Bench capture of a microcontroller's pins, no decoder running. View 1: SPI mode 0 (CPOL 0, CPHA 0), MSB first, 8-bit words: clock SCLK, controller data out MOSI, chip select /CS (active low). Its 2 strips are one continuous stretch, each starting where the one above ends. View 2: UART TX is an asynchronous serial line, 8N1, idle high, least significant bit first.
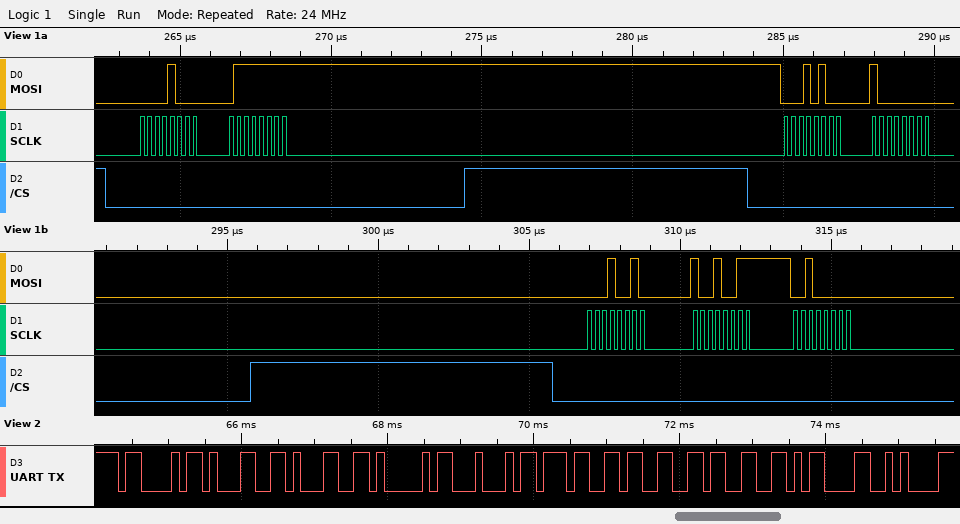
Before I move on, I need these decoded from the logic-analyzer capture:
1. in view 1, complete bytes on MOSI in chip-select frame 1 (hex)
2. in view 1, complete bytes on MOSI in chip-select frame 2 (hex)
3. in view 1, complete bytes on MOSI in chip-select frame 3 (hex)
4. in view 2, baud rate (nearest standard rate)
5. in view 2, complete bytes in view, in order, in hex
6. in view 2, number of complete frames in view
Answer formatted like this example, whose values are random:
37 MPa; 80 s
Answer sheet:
0x08 0x7F; 0x14 0x80; 0x12 0x93 0x20; 9600 baud; 43 31 31 41 44 37 33 33 0D 0A; 10
